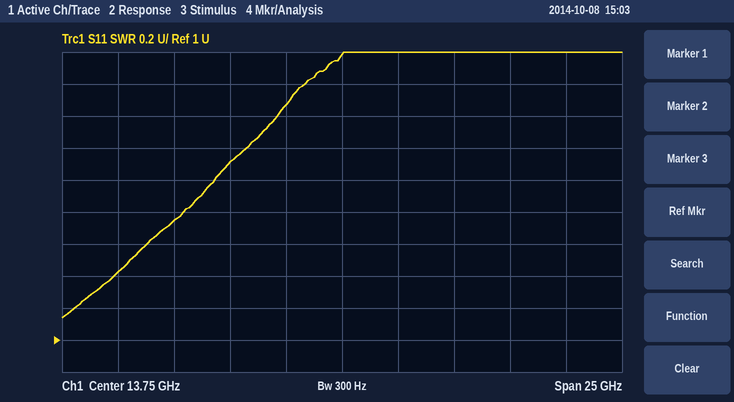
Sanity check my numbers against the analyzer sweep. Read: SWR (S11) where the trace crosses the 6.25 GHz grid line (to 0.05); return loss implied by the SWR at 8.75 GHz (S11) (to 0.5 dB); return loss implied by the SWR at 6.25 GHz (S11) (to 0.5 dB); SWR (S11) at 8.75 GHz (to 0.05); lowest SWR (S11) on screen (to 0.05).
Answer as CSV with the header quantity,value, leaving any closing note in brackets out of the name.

quantity,value
SWR (S11) where the trace crosses the 6.25 GHz grid line,1.75
return loss implied by the SWR at 8.75 GHz (S11),9.0 dB
return loss implied by the SWR at 6.25 GHz (S11),11.5 dB
SWR (S11) at 8.75 GHz,2.10
lowest SWR (S11) on screen,1.15
